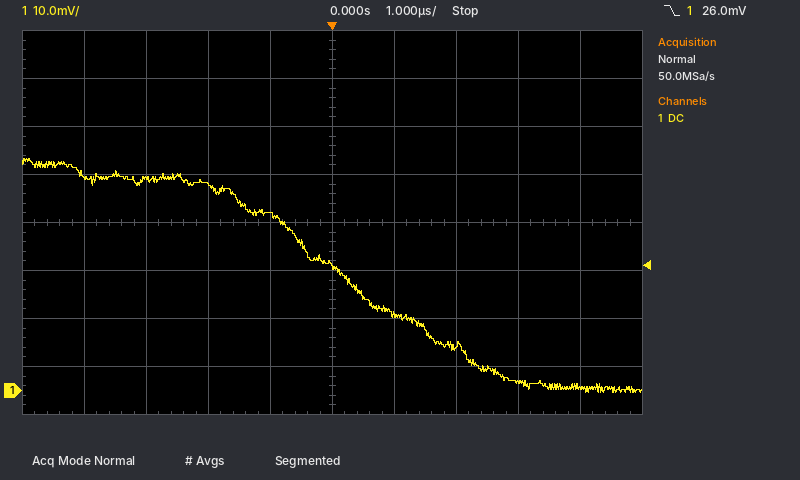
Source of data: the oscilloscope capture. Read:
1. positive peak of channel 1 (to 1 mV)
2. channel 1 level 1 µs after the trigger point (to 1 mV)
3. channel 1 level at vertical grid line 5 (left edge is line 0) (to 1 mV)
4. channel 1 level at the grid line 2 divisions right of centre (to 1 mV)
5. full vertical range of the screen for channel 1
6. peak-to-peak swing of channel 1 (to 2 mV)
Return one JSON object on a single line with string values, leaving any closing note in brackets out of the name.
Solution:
{"positive peak of channel 1": "48 mV", "channel 1 level 1 µs after the trigger point": "16 mV", "channel 1 level at vertical grid line 5 (left edge is line 0)": "26 mV", "channel 1 level at the grid line 2 divisions right of centre": "9 mV", "full vertical range of the screen for channel 1": "80 mV", "peak-to-peak swing of channel 1": "48 mV"}
